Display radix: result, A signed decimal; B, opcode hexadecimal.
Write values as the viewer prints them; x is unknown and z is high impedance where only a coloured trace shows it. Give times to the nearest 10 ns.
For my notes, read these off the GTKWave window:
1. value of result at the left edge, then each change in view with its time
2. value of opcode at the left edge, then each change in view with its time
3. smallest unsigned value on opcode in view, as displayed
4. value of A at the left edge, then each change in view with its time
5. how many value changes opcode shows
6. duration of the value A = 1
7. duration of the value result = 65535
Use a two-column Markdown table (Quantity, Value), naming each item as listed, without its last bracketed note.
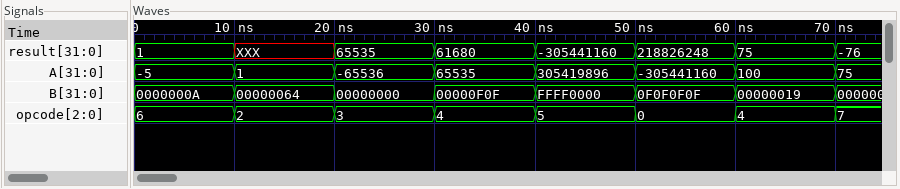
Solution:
| Quantity | Value |
|---|---|
| value of result at the left edge, then each change in view with its time | 1, XXX at 10 ns, 65535 at 20 ns, 61680 at 30 ns, -305441160 at 40 ns, 218826248 at 50 ns, 75 at 60 ns, -76 at 70 ns |
| value of opcode at the left edge, then each change in view with its time | 6, 2 at 10 ns, 3 at 20 ns, 4 at 30 ns, 5 at 40 ns, 0 at 50 ns, 4 at 60 ns, 7 at 70 ns |
| smallest unsigned value on opcode in view, as displayed | 0 |
| value of A at the left edge, then each change in view with its time | -5, 1 at 10 ns, -65536 at 20 ns, 65535 at 30 ns, 305419896 at 40 ns, -305441160 at 50 ns, 100 at 60 ns, 75 at 70 ns |
| how many value changes opcode shows | 7 |
| duration of the value A = 1 | 10 ns |
| duration of the value result = 65535 | 10 ns |
